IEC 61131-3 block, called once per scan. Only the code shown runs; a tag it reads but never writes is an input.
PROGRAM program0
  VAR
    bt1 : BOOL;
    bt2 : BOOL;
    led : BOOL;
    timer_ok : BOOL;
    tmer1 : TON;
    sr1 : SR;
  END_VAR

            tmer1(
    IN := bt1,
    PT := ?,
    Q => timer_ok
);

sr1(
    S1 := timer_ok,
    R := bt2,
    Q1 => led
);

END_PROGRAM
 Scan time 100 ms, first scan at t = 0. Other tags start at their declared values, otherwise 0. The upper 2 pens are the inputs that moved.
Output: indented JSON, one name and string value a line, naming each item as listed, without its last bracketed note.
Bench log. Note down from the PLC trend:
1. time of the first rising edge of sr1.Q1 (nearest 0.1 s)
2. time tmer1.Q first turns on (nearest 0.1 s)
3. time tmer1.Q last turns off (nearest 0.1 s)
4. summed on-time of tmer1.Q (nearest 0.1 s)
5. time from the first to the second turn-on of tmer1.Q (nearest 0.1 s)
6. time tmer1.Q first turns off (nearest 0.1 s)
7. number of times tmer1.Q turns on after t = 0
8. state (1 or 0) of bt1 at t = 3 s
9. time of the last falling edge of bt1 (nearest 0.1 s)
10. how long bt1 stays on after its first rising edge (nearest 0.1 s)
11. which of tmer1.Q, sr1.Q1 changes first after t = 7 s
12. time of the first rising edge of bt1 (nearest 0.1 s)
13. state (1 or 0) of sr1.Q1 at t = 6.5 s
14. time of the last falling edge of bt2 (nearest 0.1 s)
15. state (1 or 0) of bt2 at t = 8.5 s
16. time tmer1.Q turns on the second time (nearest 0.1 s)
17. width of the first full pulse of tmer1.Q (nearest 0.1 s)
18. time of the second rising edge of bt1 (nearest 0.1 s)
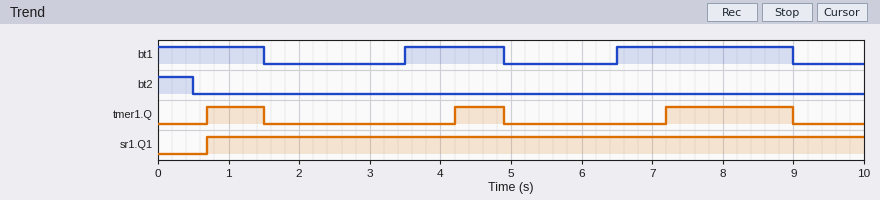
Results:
{
  "time of the first rising edge of sr1.Q1": "0.7 s",
  "time tmer1.Q first turns on": "0.7 s",
  "time tmer1.Q last turns off": "9.0 s",
  "summed on-time of tmer1.Q": "3.3 s",
  "time from the first to the second turn-on of tmer1.Q": "3.5 s",
  "time tmer1.Q first turns off": "1.5 s",
  "number of times tmer1.Q turns on after t = 0": "3",
  "state (1 or 0) of bt1 at t = 3 s": "0",
  "time of the last falling edge of bt1": "9.0 s",
  "how long bt1 stays on after its first rising edge": "1.4 s",
  "which of tmer1.Q, sr1.Q1 changes first after t = 7 s": "tmer1.Q",
  "time of the first rising edge of bt1": "3.5 s",
  "state (1 or 0) of sr1.Q1 at t = 6.5 s": "1",
  "time of the last falling edge of bt2": "0.5 s",
  "state (1 or 0) of bt2 at t = 8.5 s": "0",
  "time tmer1.Q turns on the second time": "4.2 s",
  "width of the first full pulse of tmer1.Q": "0.8 s",
  "time of the second rising edge of bt1": "6.5 s"
}
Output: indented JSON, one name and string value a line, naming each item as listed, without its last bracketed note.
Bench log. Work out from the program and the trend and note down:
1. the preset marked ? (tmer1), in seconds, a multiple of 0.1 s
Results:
{
  "the preset marked ? (tmer1), in seconds, a multiple of 0.1 s": "0.7 s"
}
